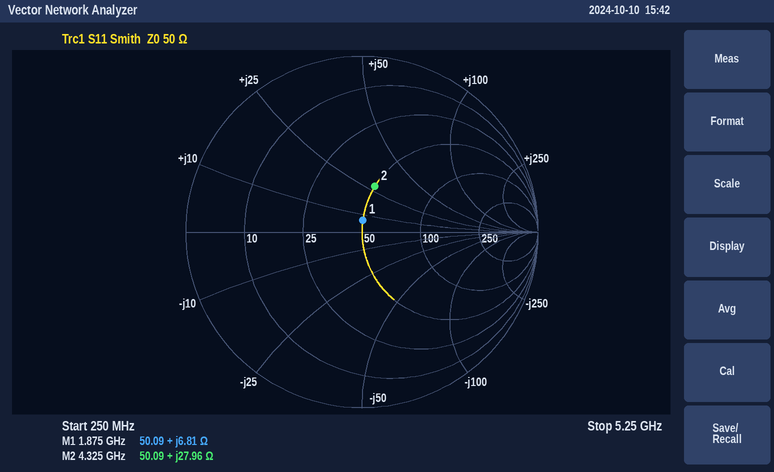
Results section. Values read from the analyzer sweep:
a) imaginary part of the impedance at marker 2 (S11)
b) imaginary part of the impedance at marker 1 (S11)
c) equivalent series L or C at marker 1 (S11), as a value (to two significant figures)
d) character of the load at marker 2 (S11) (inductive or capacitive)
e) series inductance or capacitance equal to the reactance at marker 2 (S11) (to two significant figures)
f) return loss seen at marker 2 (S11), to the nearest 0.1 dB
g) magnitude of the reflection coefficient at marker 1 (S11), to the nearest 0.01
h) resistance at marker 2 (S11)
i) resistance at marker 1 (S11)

+27.96 Ω
+6.81 Ω
580 pH
inductive
1.0 nH
11.4 dB
0.07
50.09 Ω
50.09 Ω
